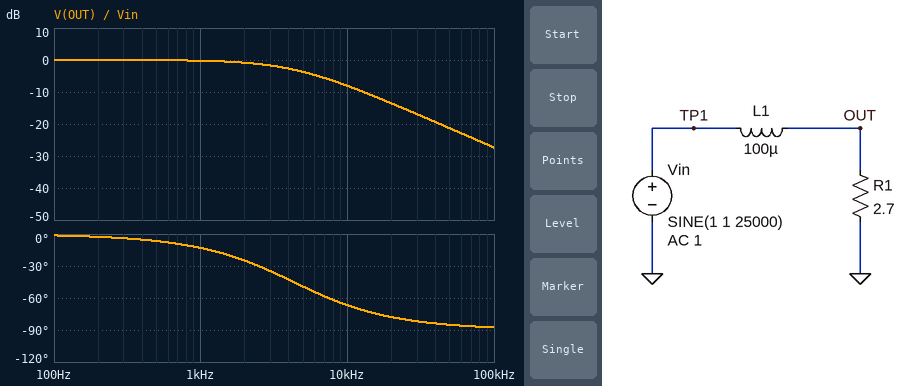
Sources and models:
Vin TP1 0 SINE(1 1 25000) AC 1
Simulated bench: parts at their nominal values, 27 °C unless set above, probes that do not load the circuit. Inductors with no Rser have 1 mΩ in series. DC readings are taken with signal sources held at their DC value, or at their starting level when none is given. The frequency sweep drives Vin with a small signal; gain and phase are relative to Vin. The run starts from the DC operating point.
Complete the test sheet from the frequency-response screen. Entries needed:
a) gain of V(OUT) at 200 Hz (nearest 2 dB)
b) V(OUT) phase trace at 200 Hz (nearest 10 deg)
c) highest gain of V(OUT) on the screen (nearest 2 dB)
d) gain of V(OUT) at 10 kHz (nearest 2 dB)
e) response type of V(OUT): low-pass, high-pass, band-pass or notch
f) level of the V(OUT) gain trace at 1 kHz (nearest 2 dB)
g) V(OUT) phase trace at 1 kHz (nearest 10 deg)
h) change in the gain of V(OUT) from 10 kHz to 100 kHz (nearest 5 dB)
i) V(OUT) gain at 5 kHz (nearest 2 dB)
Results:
0 dB
0 deg
0 dB
-8 dB
low-pass
0 dB
-10 deg
-20 dB
-4 dB
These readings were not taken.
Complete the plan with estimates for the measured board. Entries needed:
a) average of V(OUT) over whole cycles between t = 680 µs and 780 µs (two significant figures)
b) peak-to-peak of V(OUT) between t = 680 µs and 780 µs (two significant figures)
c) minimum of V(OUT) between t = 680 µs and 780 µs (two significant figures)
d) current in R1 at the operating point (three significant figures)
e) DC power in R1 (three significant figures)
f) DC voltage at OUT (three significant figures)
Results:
1.0 V
340 mV
830 mV
370 mA
370 mW
1.00 V
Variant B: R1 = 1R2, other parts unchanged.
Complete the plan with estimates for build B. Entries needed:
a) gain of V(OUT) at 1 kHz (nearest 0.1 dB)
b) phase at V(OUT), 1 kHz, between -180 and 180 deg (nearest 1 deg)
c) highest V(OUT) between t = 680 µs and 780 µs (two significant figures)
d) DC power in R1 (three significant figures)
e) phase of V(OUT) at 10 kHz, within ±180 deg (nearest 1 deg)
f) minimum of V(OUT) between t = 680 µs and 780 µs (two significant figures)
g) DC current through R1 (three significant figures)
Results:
-1.1 dB
-28 deg
1.1 V
832 mW
-79 deg
920 mV
833 mA
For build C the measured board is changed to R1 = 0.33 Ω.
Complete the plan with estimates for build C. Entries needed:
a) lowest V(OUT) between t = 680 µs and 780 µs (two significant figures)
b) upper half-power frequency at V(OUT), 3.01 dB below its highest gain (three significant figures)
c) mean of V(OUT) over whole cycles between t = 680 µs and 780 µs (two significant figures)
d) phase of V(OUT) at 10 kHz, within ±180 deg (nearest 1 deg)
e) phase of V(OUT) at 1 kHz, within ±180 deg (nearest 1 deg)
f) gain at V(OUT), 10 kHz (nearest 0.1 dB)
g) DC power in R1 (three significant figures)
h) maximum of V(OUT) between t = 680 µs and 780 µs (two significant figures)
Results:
980 mV
527 Hz
1.0 V
-87 deg
-62 deg
-25.6 dB
3.01 W
1.0 V
